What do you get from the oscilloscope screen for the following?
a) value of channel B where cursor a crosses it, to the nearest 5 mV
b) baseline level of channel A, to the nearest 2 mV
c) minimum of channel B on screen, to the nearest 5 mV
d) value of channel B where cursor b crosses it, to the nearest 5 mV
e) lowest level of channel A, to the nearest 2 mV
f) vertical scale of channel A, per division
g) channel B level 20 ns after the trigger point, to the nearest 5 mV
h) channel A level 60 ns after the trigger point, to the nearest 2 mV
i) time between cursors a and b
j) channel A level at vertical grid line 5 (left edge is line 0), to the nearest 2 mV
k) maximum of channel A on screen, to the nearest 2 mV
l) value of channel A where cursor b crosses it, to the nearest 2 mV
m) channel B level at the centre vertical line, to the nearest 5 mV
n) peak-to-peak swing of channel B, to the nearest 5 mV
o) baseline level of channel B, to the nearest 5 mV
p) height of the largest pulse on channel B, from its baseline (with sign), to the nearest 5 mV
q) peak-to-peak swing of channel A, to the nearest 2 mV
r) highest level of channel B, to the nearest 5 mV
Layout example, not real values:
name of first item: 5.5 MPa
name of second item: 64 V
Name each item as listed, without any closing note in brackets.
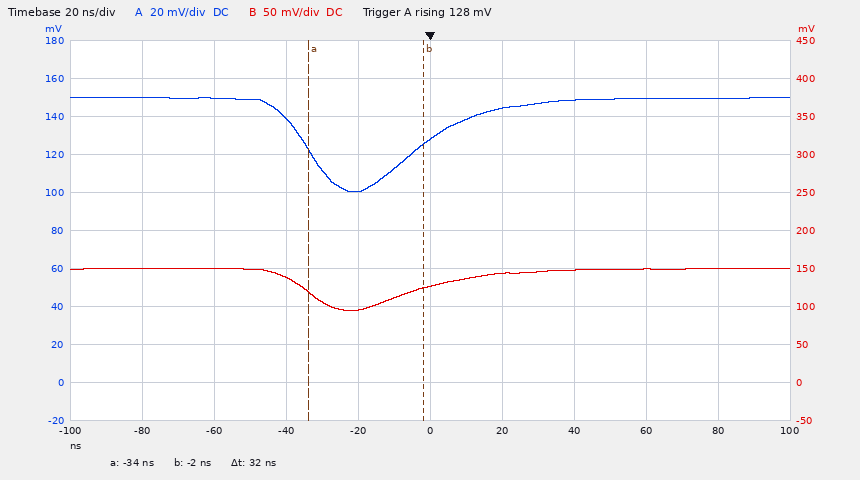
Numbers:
value of channel B where cursor a crosses it, to the nearest 5 mV: 120 mV
baseline level of channel A, to the nearest 2 mV: 150 mV
minimum of channel B on screen, to the nearest 5 mV: 95 mV
value of channel B where cursor b crosses it, to the nearest 5 mV: 125 mV
lowest level of channel A, to the nearest 2 mV: 100 mV
vertical scale of channel A, per division: 20 mV
channel B level 20 ns after the trigger point, to the nearest 5 mV: 145 mV
channel A level 60 ns after the trigger point, to the nearest 2 mV: 150 mV
time between cursors a and b: 32 ns
channel A level at vertical grid line 5 (left edge is line 0), to the nearest 2 mV: 128 mV
maximum of channel A on screen, to the nearest 2 mV: 150 mV
value of channel A where cursor b crosses it, to the nearest 2 mV: 126 mV
channel B level at the centre vertical line, to the nearest 5 mV: 125 mV
peak-to-peak swing of channel B, to the nearest 5 mV: 55 mV
baseline level of channel B, to the nearest 5 mV: 150 mV
height of the largest pulse on channel B, from its baseline (with sign), to the nearest 5 mV: -55 mV
peak-to-peak swing of channel A, to the nearest 2 mV: 50 mV
highest level of channel B, to the nearest 5 mV: 150 mV
